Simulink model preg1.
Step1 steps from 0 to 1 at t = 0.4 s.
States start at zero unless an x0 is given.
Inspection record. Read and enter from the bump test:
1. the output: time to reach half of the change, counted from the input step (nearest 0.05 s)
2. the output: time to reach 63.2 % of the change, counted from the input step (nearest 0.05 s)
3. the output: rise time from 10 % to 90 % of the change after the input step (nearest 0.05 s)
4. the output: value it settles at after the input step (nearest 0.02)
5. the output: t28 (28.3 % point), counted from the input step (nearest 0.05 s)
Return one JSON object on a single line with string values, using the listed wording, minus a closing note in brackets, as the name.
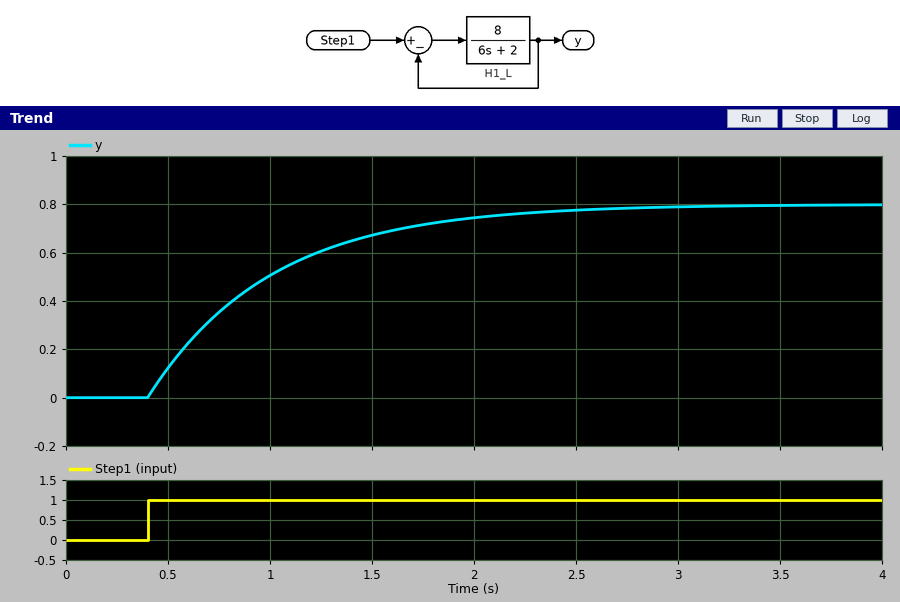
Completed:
{"the output: time to reach half of the change, counted from the input step": "0.40 s", "the output: time to reach 63.2 % of the change, counted from the input step": "0.60 s", "the output: rise time from 10 % to 90 % of the change after the input step": "1.30 s", "the output: value it settles at after the input step": "0.80", "the output: t28 (28.3 % point), counted from the input step": "0.20 s"}
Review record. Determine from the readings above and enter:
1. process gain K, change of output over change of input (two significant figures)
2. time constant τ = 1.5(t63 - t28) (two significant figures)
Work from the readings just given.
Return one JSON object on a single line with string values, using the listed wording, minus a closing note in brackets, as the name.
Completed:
{"process gain K, change of output over change of input": "0.80", "time constant τ = 1.5(t63 - t28)": "0.60 s"}
